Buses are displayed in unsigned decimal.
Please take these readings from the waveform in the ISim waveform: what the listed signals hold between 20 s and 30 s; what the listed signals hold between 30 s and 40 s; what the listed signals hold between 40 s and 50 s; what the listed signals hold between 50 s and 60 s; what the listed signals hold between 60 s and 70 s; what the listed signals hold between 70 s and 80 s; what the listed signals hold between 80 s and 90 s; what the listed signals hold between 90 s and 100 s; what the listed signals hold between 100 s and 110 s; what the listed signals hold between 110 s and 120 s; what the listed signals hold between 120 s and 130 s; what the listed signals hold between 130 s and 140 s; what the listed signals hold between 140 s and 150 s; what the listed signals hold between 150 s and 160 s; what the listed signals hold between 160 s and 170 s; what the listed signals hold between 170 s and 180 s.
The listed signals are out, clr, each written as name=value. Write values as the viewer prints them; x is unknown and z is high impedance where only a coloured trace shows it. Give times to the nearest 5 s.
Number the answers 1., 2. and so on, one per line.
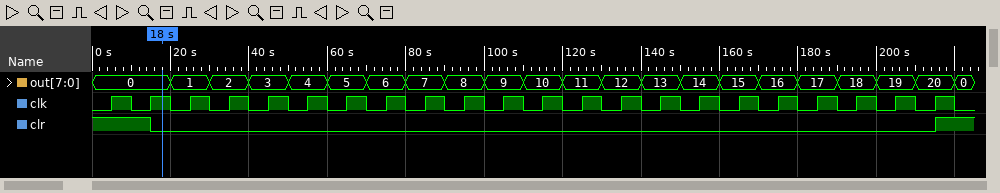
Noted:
1. out=1, clr=0
2. out=2, clr=0
3. out=3, clr=0
4. out=4, clr=0
5. out=5, clr=0
6. out=6, clr=0
7. out=7, clr=0
8. out=8, clr=0
9. out=9, clr=0
10. out=10, clr=0
11. out=11, clr=0
12. out=12, clr=0
13. out=13, clr=0
14. out=14, clr=0
15. out=15, clr=0
16. out=16, clr=0
